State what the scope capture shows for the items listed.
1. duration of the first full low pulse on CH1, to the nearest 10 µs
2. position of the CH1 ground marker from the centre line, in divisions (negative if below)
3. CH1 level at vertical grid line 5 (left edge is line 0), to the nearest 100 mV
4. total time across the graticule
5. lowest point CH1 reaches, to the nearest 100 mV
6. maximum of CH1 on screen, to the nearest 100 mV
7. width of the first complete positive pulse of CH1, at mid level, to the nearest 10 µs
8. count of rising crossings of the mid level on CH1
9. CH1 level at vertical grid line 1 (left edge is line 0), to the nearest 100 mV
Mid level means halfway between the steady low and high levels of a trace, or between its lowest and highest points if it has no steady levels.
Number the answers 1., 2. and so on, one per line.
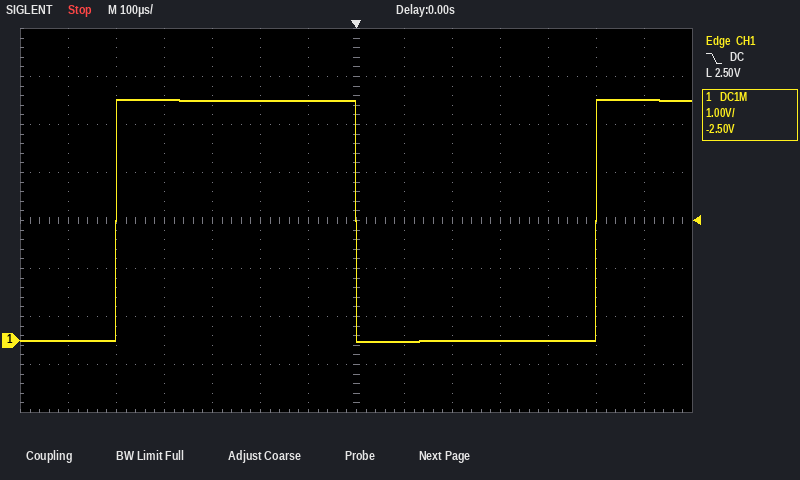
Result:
1. 500 µs
2. -2.5 div
3. 5.0 V
4. 1.4 ms
5. 0.0 V
6. 5.0 V
7. 500 µs
8. 2
9. 0.0 V
